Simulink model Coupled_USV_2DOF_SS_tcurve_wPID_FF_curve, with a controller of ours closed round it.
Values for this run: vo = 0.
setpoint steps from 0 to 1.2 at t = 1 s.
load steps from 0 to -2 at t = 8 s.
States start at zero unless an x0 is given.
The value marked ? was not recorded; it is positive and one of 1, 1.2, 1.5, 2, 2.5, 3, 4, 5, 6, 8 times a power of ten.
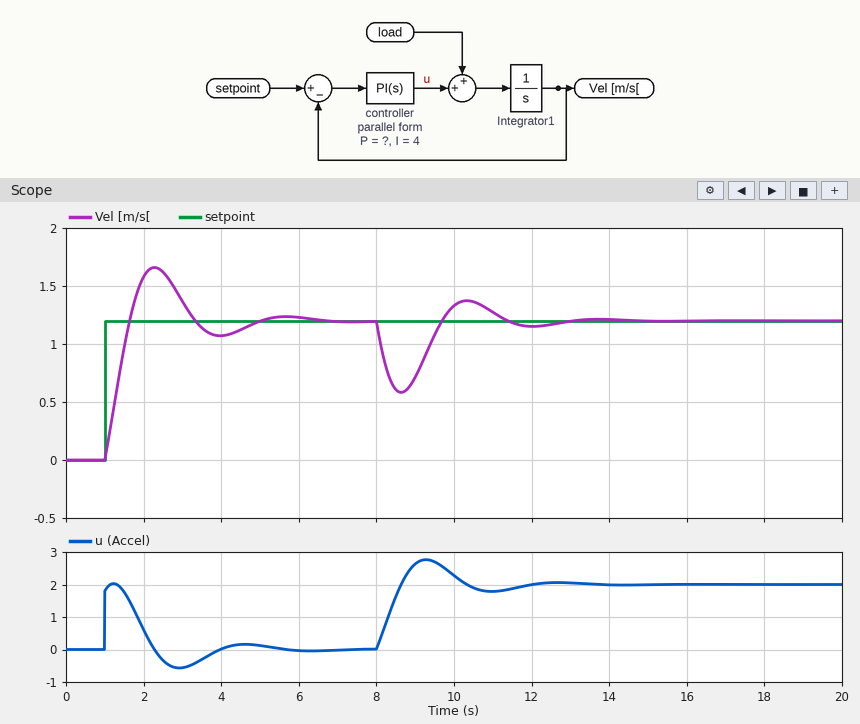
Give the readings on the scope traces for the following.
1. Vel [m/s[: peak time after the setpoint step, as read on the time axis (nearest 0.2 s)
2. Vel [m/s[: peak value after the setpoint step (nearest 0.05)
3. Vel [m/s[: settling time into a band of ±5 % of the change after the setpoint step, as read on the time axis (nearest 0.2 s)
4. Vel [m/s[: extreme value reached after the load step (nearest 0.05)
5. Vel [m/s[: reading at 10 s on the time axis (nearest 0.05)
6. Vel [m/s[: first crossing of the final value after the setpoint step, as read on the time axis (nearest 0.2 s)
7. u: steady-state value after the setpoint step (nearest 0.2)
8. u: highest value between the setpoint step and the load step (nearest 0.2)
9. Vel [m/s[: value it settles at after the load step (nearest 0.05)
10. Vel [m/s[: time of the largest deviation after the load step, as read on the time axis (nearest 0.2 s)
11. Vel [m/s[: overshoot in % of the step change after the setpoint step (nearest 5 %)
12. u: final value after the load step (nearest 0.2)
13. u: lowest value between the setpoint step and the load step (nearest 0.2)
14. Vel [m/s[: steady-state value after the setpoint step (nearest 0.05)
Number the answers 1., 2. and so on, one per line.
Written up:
1. 2.2 s
2. 1.65
3. 4.6 s
4. 0.60
5. 1.35
6. 1.6 s
7. 0.0
8. 2.0
9. 1.20
10. 8.6 s
11. 40 %
12. 2.0
13. -0.6
14. 1.20
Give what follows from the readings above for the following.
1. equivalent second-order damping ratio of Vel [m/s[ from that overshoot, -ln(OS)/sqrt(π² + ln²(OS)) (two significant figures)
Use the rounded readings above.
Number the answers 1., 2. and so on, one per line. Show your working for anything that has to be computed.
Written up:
1. ln(0.4) = -0.916; 0.916 / sqrt(9.870 + 0.840) = 0.28
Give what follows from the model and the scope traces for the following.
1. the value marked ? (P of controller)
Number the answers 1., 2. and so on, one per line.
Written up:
1. 1.5
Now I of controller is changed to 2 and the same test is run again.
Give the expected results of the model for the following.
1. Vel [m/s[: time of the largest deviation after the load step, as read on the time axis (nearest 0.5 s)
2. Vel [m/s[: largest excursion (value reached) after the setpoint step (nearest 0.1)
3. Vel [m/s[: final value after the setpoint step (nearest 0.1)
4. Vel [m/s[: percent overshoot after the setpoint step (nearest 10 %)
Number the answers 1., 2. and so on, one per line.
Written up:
1. 9.0 s
2. 1.5
3. 1.2
4. 30 %
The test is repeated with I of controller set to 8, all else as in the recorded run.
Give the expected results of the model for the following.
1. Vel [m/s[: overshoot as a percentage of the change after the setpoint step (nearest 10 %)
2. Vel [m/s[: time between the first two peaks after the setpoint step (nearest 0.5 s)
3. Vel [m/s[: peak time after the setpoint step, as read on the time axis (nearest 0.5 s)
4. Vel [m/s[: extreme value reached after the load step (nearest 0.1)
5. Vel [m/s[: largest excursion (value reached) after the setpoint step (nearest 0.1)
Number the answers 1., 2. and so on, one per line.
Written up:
1. 50 %
2. 2.5 s
3. 2.0 s
4. 0.7
5. 1.8
